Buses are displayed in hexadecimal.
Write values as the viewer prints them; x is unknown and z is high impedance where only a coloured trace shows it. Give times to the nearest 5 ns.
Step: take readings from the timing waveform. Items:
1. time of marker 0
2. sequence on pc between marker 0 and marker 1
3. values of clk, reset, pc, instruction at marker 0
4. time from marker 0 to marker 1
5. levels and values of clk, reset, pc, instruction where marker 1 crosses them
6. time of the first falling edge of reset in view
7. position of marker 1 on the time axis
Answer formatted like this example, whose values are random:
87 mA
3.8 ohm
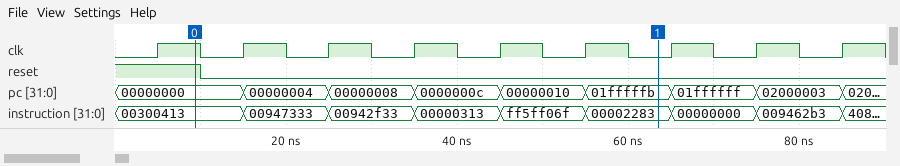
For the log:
10 ns
00000000, 00000004, 00000008, 0000000c, 00000010, 01fffffb
clk=1, reset=1, pc=00000000, instruction=00300413
55 ns
clk=0, reset=0, pc=01fffffb, instruction=00002283
10 ns
65 ns
